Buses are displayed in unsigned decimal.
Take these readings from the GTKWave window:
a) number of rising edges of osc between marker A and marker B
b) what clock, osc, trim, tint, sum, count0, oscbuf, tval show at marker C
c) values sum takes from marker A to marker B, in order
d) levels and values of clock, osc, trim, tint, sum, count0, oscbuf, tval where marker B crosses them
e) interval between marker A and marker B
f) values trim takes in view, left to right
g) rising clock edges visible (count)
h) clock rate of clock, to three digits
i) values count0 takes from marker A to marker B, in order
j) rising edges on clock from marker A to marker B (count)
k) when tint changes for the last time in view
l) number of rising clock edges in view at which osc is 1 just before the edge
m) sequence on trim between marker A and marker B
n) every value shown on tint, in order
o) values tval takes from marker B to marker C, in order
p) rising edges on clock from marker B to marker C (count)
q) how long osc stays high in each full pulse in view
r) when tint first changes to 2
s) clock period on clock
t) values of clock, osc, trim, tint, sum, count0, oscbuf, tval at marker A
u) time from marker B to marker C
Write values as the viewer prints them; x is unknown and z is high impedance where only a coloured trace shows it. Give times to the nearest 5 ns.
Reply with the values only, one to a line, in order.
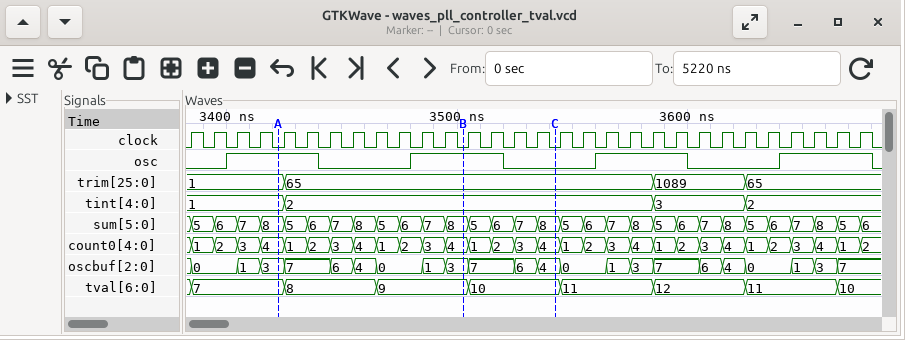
1
clock=0, osc=0, trim=65, tint=2, sum=8, count0=4, oscbuf=4, tval=10
8, 5, 6, 7, 8, 5, 6, 7, 8
clock=0, osc=1, trim=65, tint=2, sum=8, count0=4, oscbuf=3, tval=9
80 ns
1, 65, 1089, 65
30
100 MHz
4, 1, 2, 3, 4, 1, 2, 3, 4
8
3625 ns
16
1, 65
1, 2, 3, 2
9, 10
4
40 ns, 40 ns, 40 ns, 40 ns
3425 ns
10 ns
clock=0, osc=1, trim=1, tint=1, sum=8, count0=4, oscbuf=3, tval=7
40 ns
